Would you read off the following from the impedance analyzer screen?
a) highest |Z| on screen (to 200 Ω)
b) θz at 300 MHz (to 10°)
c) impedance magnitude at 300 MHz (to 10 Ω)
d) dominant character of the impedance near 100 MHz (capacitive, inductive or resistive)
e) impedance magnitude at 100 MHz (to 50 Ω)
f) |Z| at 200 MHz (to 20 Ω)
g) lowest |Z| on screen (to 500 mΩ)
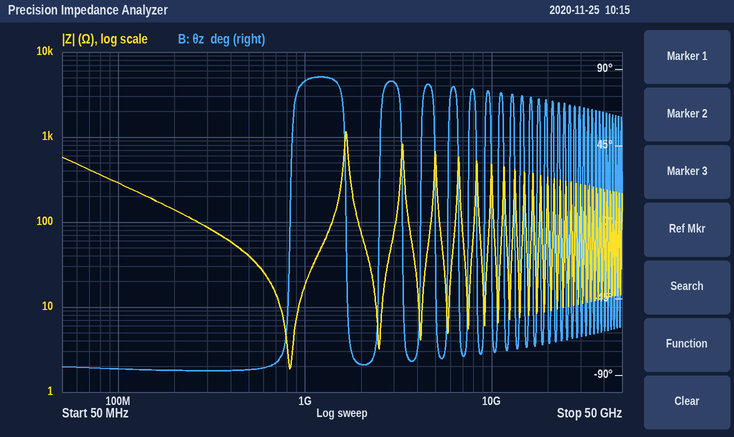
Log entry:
1.2 kΩ
-90°
90 Ω
capacitive
300 Ω
140 Ω
2.0 Ω
